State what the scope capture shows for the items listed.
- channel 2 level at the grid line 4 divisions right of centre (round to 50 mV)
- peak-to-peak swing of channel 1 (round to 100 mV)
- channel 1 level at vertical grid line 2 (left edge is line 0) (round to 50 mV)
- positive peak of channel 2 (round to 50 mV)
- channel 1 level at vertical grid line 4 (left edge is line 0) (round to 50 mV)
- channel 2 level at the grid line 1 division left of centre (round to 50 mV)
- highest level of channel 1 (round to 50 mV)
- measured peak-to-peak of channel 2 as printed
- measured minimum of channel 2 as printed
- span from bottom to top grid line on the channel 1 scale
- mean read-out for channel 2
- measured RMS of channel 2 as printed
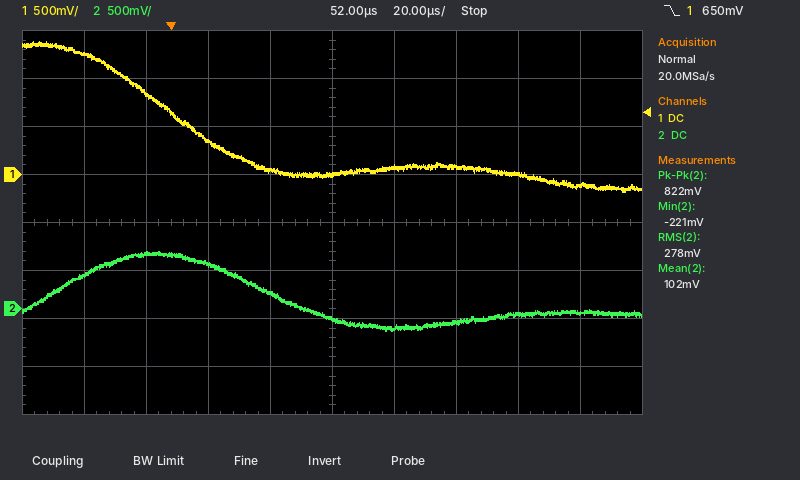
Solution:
-50 mV
1.60 V
850 mV
600 mV
50 mV
150 mV
1.40 V
822 mV
-221 mV
4 V
102 mV
278 mV
